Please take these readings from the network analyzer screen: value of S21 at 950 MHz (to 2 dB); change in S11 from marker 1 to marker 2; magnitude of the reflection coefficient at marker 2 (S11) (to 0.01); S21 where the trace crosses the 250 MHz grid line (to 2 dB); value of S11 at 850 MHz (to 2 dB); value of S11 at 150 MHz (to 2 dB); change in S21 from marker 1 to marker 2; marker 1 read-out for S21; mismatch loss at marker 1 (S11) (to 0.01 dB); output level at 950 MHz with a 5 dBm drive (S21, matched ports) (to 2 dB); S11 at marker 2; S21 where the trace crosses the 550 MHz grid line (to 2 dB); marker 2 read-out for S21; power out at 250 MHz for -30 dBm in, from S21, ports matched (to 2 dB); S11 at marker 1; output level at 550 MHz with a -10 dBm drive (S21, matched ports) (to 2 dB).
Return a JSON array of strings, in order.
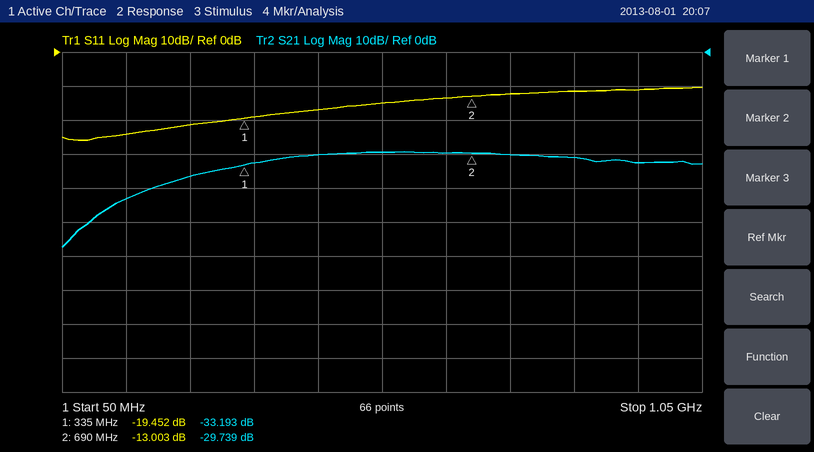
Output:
["-32 dB", "6.449 dB", "0.22", "-36 dB", "-12 dB", "-24 dB", "3.454 dB", "-33.193 dB", "0.05 dB", "-28 dBm", "-13.003 dB", "-30 dB", "-29.739 dB", "-66 dBm", "-19.452 dB", "-40 dBm"]
